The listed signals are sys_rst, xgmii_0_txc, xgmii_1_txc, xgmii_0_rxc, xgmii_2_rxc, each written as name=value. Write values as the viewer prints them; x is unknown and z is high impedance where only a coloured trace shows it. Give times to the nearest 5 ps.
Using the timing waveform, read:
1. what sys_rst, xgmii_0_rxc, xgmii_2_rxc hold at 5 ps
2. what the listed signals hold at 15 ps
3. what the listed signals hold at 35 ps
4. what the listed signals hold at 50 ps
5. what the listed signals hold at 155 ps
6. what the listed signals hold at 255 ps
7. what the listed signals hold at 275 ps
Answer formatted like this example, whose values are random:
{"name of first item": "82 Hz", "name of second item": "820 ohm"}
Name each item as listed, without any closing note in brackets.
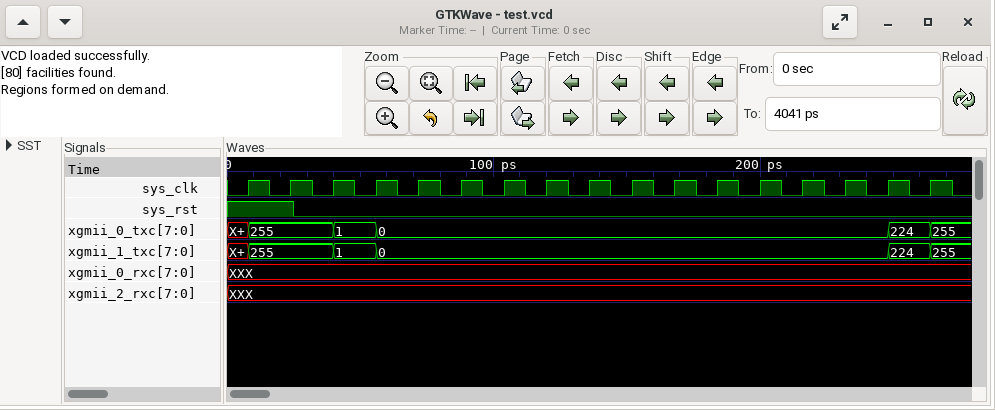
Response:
{"what sys_rst, xgmii_0_rxc, xgmii_2_rxc hold at 5 ps": "sys_rst=1, xgmii_0_rxc=XXX, xgmii_2_rxc=XXX", "what the listed signals hold at 15 ps": "sys_rst=1, xgmii_0_txc=255, xgmii_1_txc=255, xgmii_0_rxc=XXX, xgmii_2_rxc=XXX", "what the listed signals hold at 35 ps": "sys_rst=0, xgmii_0_txc=255, xgmii_1_txc=255, xgmii_0_rxc=XXX, xgmii_2_rxc=XXX", "what the listed signals hold at 50 ps": "sys_rst=0, xgmii_0_txc=1, xgmii_1_txc=1, xgmii_0_rxc=XXX, xgmii_2_rxc=XXX", "what the listed signals hold at 155 ps": "sys_rst=0, xgmii_0_txc=0, xgmii_1_txc=0, xgmii_0_rxc=XXX, xgmii_2_rxc=XXX", "what the listed signals hold at 255 ps": "sys_rst=0, xgmii_0_txc=224, xgmii_1_txc=224, xgmii_0_rxc=XXX, xgmii_2_rxc=XXX", "what the listed signals hold at 275 ps": "sys_rst=0, xgmii_0_txc=255, xgmii_1_txc=255, xgmii_0_rxc=XXX, xgmii_2_rxc=XXX"}
